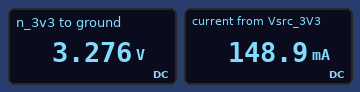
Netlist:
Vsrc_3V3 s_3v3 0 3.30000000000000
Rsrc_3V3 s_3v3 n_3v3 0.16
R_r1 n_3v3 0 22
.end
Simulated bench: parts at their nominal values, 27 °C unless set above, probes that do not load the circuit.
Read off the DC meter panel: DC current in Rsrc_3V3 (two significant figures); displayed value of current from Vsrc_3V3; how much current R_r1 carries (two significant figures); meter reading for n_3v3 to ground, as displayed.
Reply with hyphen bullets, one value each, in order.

- 150 mA
- 148.9 mA
- 150 mA
- 3.276 V
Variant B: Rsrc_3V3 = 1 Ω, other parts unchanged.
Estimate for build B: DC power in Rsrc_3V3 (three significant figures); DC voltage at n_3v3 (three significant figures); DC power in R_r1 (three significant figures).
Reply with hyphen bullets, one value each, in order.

- 20.6 mW
- 3.16 V
- 453 mW
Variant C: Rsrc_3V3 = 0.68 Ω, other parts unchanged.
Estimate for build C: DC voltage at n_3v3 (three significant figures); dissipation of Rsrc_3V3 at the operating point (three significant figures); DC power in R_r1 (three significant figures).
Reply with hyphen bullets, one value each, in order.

- 3.20 V
- 14.4 mW
- 466 mW
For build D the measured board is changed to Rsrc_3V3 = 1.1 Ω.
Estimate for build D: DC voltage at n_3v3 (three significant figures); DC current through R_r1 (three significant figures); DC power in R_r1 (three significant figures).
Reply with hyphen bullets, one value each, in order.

- 3.14 V
- 143 mA
- 449 mW
